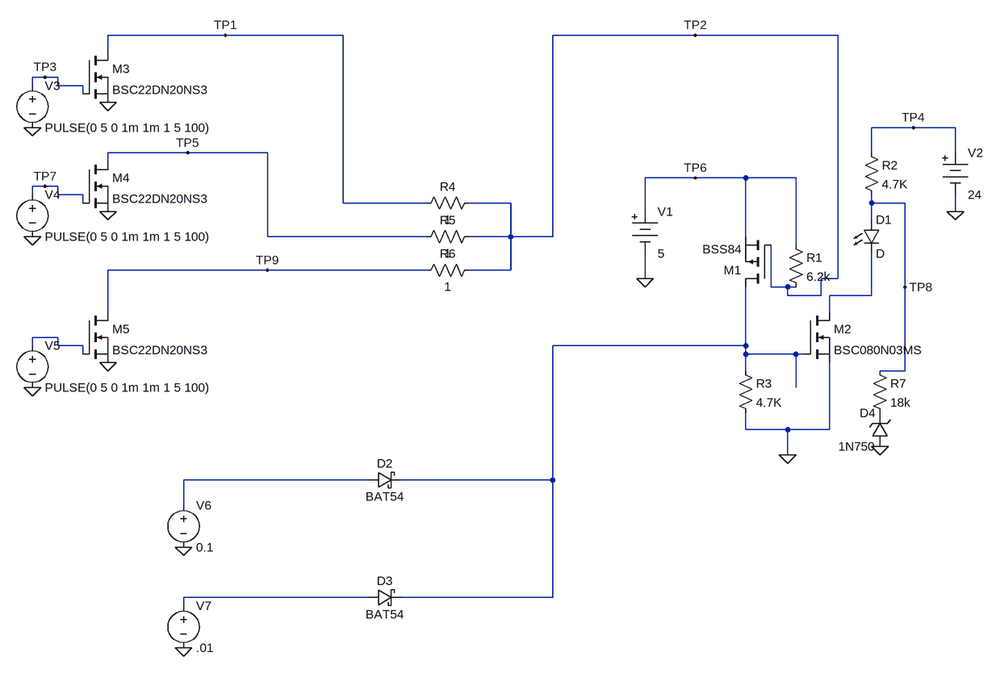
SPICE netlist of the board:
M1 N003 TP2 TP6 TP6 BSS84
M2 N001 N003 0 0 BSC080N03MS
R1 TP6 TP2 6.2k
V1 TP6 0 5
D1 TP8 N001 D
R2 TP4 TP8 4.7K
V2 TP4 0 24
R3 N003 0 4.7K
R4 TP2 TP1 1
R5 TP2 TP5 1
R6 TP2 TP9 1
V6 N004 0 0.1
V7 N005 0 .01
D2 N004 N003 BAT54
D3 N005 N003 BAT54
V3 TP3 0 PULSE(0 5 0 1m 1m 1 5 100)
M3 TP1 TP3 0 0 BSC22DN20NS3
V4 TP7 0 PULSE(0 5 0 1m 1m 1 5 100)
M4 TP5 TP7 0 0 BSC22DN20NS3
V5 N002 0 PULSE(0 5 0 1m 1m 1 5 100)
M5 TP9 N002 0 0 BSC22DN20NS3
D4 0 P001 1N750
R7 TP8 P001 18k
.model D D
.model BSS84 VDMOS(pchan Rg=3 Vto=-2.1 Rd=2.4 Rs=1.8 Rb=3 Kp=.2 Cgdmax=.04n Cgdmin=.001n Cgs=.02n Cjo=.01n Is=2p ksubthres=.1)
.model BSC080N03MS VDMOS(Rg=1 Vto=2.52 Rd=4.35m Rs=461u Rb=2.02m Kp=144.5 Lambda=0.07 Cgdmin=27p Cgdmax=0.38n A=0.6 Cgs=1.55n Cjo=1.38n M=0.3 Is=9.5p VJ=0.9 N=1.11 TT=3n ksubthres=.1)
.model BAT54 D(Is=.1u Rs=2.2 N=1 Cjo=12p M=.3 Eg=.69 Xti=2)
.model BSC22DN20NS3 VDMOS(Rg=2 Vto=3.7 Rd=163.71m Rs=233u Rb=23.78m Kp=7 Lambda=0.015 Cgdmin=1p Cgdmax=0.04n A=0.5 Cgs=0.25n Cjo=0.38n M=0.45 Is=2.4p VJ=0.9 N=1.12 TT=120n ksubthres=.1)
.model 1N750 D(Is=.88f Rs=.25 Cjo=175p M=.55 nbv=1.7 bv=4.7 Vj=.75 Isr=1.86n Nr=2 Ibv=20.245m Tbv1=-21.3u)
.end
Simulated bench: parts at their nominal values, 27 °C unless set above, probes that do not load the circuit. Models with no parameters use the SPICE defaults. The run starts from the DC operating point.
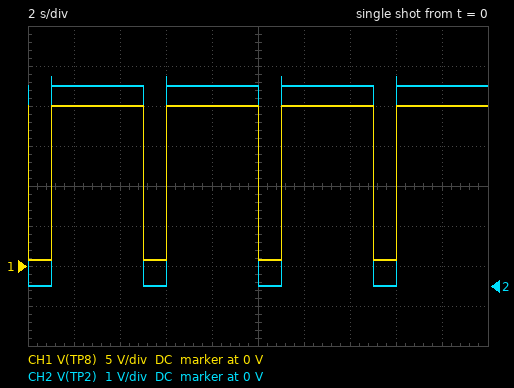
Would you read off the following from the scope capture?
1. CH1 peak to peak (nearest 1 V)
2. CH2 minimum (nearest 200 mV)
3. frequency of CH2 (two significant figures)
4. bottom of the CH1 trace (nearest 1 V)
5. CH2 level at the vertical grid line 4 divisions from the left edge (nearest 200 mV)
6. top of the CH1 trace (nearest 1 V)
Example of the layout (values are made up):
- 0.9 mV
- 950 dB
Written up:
- 19 V
- 0 V
- 200 mHz
- 1 V
- 5.0 V
- 20 V
